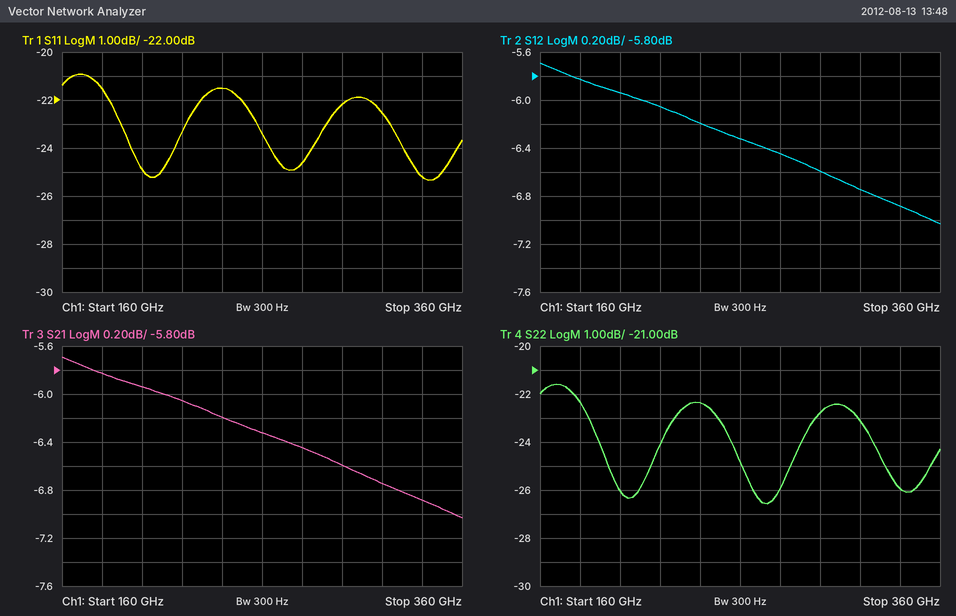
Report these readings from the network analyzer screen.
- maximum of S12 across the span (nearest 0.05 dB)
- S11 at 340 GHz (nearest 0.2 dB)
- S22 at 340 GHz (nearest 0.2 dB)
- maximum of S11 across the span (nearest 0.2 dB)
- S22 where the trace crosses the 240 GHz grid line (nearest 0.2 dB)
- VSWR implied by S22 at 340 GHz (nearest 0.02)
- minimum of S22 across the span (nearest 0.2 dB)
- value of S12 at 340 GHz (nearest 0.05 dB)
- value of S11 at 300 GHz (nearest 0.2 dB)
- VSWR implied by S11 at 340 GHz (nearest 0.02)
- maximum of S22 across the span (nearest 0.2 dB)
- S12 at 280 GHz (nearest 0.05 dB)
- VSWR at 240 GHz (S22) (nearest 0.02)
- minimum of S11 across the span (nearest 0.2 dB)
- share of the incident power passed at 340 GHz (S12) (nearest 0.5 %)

-5.70 dB
-25.2 dB
-26.0 dB
-21.0 dB
-22.4 dB
1.10
-26.6 dB
-6.90 dB
-22.2 dB
1.12
-21.6 dB
-6.45 dB
1.16
-25.4 dB
20.5 %
